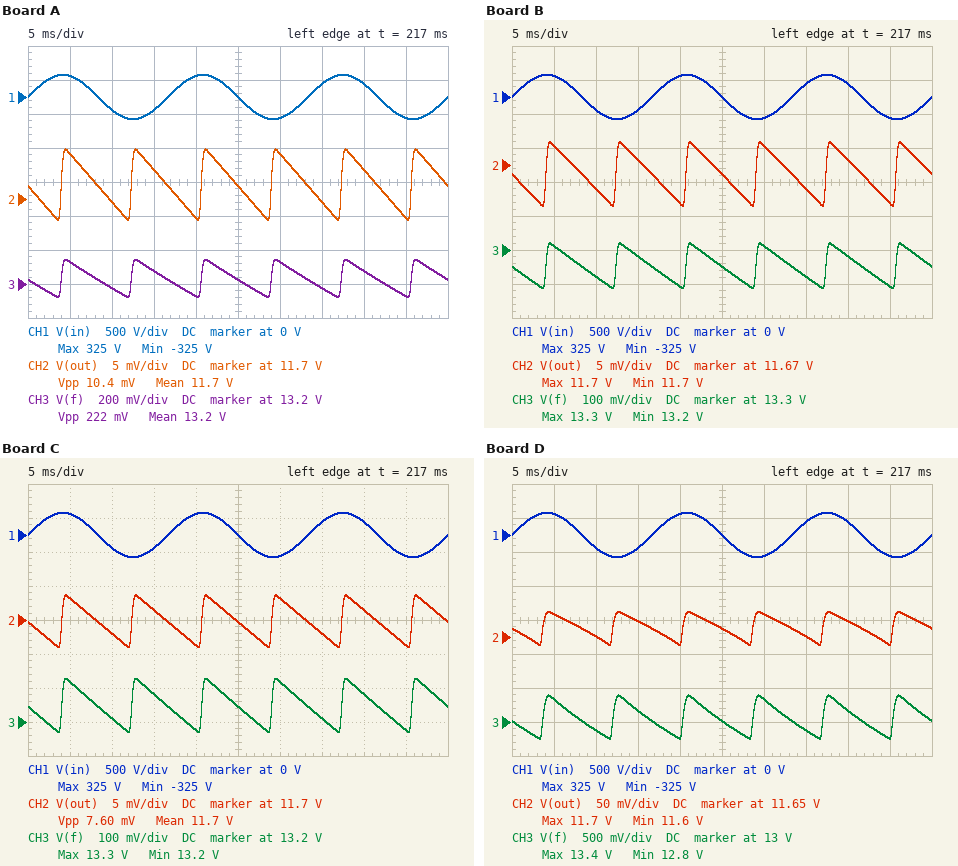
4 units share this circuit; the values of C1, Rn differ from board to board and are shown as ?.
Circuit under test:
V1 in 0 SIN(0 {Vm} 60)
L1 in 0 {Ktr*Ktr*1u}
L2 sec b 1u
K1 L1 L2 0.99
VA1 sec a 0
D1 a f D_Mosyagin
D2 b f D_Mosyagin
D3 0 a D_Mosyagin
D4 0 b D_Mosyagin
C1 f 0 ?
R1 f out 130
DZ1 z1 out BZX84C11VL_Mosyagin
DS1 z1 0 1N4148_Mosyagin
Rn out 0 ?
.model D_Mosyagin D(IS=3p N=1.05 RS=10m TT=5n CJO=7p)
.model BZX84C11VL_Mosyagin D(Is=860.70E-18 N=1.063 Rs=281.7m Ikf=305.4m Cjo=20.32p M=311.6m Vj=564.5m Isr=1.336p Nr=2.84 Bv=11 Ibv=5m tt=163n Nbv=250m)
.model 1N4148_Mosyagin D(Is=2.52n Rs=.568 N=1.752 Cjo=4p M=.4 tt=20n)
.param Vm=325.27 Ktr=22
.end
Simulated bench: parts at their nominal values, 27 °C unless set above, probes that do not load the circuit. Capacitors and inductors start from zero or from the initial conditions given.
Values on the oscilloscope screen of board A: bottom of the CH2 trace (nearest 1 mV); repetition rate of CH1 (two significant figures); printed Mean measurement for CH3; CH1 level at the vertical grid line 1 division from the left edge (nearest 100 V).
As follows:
11.692 V
60 Hz
13.2 V
300 V
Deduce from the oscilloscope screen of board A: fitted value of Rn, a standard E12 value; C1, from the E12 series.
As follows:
4.7 kΩ
390 µF
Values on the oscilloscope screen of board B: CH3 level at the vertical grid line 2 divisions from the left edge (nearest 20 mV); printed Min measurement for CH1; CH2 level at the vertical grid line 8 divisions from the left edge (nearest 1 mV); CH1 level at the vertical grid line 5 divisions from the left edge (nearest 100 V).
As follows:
13.22 V
-325 V
11.671 V
0 V
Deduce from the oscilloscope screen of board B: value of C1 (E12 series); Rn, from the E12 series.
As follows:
680 µF
1.8 kΩ
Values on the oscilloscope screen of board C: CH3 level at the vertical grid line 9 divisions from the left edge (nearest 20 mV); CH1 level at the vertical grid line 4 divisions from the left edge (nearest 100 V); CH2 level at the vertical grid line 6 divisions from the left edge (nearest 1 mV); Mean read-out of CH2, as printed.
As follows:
13.18 V
300 V
11.698 V
11.7 V
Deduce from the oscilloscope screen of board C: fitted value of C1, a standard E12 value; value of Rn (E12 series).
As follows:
560 µF
3.9 kΩ
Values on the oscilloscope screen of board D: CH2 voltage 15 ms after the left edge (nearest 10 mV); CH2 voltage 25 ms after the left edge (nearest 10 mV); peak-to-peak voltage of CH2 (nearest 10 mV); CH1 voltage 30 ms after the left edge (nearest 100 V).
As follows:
11.67 V
11.66 V
50 mV
-300 V
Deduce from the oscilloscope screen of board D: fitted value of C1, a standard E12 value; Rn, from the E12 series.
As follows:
120 µF
2.2 kΩ
